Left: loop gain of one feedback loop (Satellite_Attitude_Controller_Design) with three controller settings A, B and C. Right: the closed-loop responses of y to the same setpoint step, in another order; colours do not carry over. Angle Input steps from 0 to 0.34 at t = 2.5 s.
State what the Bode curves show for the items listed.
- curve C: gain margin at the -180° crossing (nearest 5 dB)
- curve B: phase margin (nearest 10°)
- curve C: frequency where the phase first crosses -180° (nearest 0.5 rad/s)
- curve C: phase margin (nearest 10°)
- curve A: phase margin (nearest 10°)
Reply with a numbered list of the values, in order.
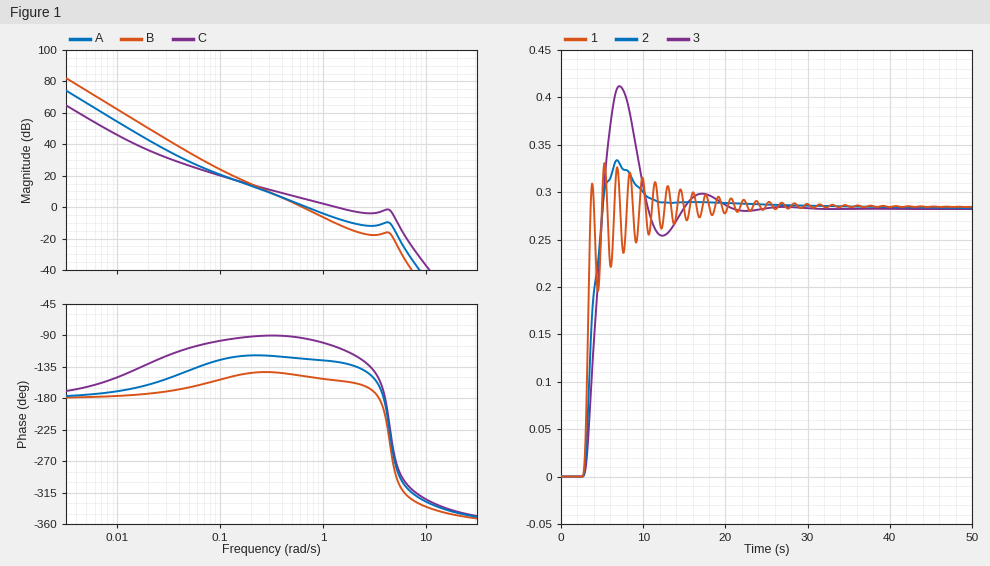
1. 0 dB
2. 30°
3. 4.0 rad/s
4. 70°
5. 60°
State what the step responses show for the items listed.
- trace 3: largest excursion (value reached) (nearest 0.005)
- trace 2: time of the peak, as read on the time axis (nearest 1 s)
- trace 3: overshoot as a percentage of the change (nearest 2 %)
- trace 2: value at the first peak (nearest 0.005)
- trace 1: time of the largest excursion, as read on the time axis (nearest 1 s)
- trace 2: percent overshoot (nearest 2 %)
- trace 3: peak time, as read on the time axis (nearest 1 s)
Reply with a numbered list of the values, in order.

1. 0.410
2. 7 s
3. 46 %
4. 0.335
5. 5 s
6. 18 %
7. 7 s
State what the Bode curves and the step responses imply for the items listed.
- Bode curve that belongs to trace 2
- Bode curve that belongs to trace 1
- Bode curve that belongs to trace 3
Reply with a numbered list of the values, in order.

1. A
2. C
3. B
